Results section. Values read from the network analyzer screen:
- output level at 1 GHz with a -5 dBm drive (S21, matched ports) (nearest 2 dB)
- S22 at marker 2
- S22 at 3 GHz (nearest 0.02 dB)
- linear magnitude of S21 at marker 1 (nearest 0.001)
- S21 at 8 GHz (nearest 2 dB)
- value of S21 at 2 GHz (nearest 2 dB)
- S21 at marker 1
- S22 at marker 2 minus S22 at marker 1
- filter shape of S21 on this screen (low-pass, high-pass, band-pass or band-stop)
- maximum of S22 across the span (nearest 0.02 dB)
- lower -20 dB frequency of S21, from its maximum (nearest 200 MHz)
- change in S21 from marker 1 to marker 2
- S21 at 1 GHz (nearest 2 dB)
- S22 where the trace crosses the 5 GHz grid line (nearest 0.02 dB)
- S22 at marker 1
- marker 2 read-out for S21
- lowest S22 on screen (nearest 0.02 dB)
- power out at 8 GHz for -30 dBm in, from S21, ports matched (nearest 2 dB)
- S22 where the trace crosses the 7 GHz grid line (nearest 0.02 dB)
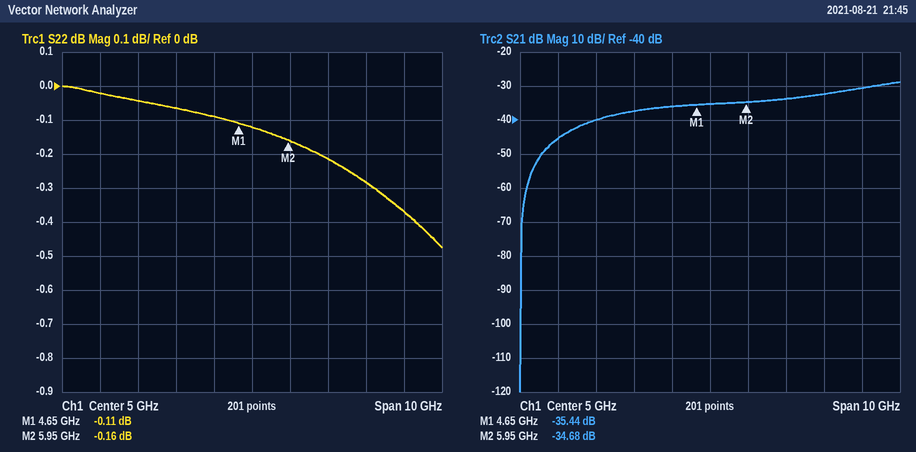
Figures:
-50 dBm
-0.16 dB
-0.06 dB
0.017
-32 dB
-40 dB
-35.44 dB
-0.05 dB
high-pass
0.00 dB
600 MHz
0.76 dB
-46 dB
-0.12 dB
-0.11 dB
-34.68 dB
-0.48 dB
-62 dBm
-0.22 dB
